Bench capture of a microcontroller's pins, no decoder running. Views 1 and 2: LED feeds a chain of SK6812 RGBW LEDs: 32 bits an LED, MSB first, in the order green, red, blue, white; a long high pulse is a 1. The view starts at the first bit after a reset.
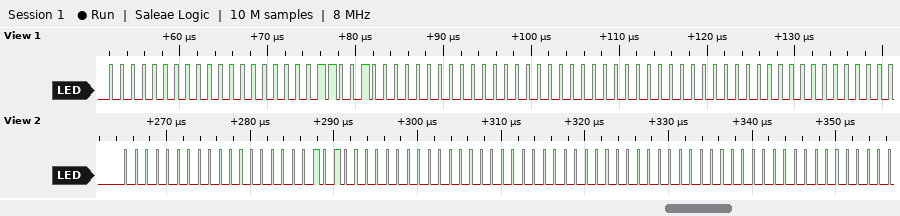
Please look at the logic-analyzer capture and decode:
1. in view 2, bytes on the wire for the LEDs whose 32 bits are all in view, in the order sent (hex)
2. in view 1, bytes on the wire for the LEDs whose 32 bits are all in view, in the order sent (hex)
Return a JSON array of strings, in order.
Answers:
["00 00 28 00 00 00 00 00", "00 00 19 00 00 00 00 00"]
